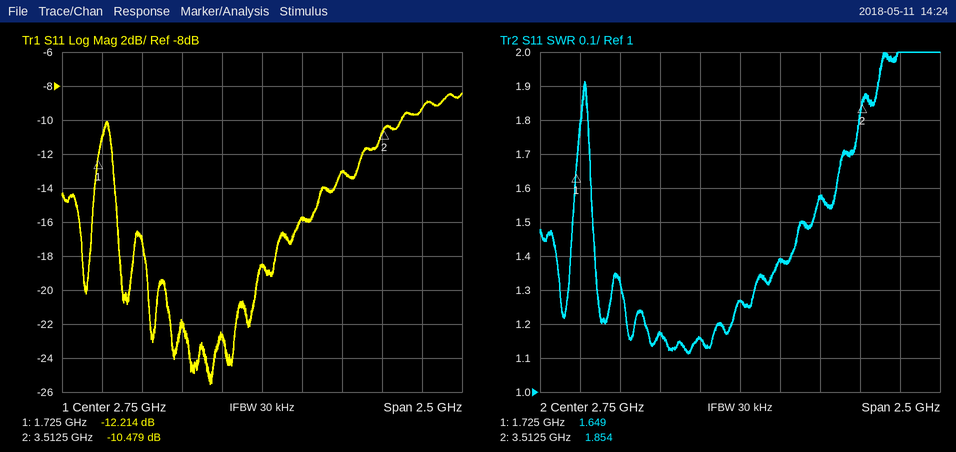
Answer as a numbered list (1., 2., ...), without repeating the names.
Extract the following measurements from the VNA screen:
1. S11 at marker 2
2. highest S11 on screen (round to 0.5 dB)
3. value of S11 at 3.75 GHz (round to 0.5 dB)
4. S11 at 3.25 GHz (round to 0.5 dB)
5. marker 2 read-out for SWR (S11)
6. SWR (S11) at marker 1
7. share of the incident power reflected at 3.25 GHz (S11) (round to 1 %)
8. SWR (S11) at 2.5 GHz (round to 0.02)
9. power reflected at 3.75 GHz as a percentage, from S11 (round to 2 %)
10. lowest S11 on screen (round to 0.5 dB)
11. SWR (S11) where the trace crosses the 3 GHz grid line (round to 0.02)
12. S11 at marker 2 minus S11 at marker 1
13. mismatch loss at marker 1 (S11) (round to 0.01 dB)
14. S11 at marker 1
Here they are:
1. -10.479 dB
2. -8.5 dB
3. -9.5 dB
4. -13.0 dB
5. 1.854
6. 1.649
7. 5 %
8. 1.16
9. 12 %
10. -25.5 dB
11. 1.38
12. 1.735 dB
13. 0.27 dB
14. -12.214 dB
